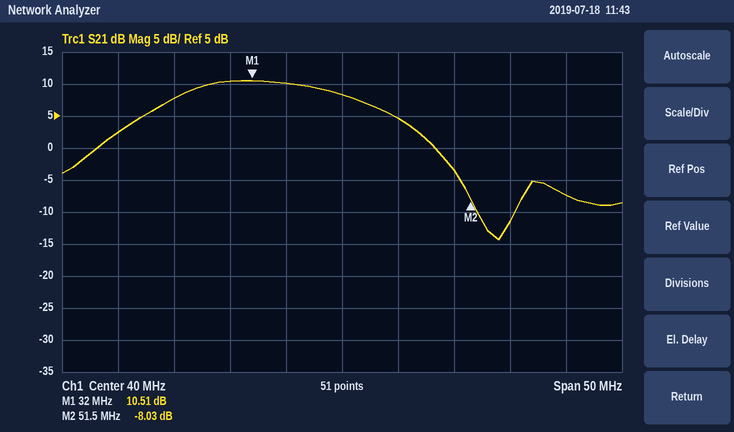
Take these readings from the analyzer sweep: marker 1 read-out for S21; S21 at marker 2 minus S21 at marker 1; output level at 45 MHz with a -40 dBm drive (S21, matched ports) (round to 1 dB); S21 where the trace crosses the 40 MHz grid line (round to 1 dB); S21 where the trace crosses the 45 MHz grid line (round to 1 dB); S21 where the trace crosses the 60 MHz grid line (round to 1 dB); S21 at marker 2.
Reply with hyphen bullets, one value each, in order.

- 10.51 dB
- -18.54 dB
- -35 dBm
- 8 dB
- 5 dB
- -7 dB
- -8.03 dB
